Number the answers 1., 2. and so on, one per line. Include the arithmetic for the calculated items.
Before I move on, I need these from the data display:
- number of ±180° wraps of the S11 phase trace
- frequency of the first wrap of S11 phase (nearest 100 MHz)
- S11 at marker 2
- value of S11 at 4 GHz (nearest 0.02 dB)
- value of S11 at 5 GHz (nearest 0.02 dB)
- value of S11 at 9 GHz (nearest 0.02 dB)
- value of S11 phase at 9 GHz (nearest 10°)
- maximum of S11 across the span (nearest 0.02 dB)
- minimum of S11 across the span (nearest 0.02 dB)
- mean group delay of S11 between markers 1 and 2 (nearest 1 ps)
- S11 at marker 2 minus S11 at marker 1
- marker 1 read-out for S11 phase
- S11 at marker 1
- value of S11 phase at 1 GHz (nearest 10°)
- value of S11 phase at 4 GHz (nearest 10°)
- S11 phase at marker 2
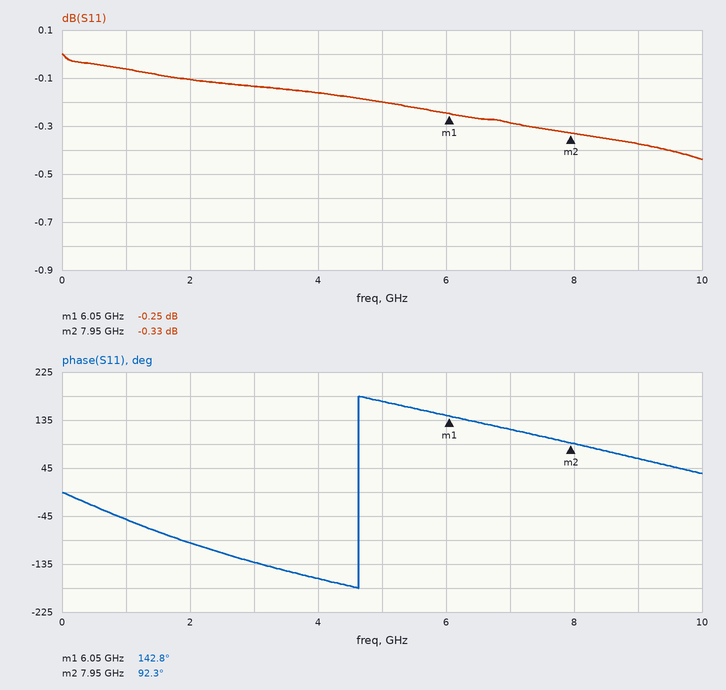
1. 1
2. 4.6 GHz
3. -0.33 dB
4. -0.16 dB
5. -0.20 dB
6. -0.38 dB
7. 60°
8. 0.00 dB
9. -0.44 dB
10. −(92.3° − (142.8°))/(360° × 1.9 GHz) ≈ 74 ps
11. -0.33 − (-0.25) = -0.08 dB
12. 142.8°
13. -0.25 dB
14. -50°
15. -160°
16. 92.3°
